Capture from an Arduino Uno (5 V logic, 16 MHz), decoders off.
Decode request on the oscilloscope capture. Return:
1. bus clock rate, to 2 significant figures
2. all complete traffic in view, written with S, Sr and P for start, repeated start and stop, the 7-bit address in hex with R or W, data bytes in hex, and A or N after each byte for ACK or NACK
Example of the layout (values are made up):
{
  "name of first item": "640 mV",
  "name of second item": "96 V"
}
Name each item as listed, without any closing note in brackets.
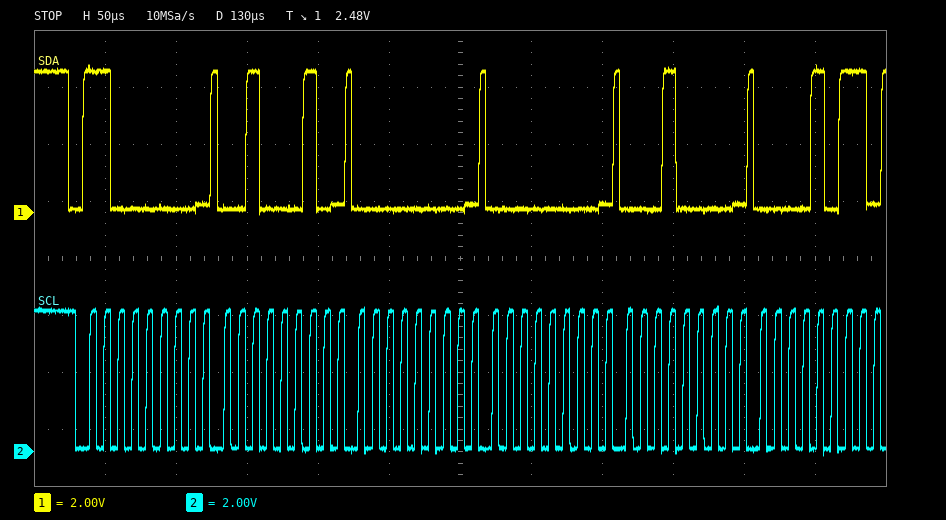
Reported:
{
  "bus clock rate, to 2 significant figures": "100 kHz",
  "all complete traffic in view, written with S, Sr and P for start, repeated start and stop, the 7-bit address in hex with R or W, data bytes in hex, and A or N after each byte for ACK or NACK": "S 60W A 22 A 00 A 00 A 10 A 0B A"
}
